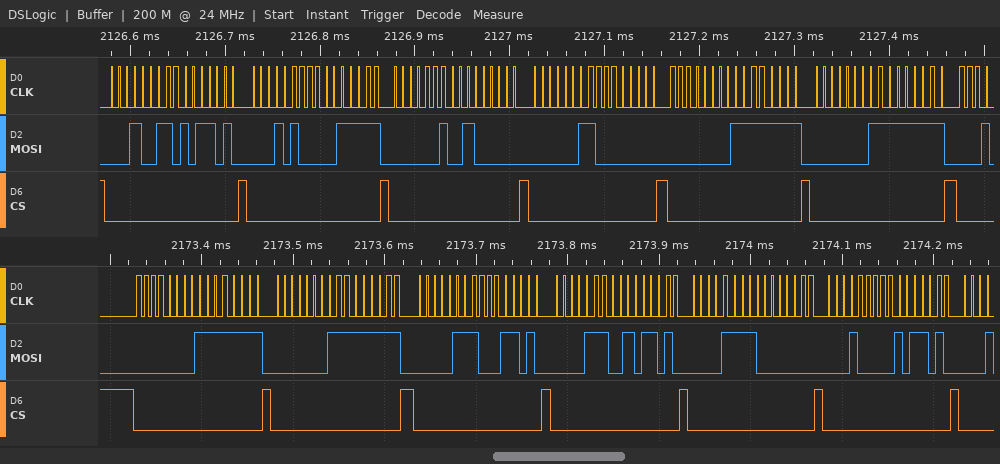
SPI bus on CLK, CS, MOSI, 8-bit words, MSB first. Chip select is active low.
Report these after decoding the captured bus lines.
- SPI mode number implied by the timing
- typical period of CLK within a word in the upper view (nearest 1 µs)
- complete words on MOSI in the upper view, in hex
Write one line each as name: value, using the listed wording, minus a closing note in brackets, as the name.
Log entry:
SPI mode number implied by the timing: 1
typical period of CLK within a word in the upper view: 8 µs
complete words on MOSI in the upper view, in hex: 13, 5A, 14, 1F, 02, 40, 03, 00, 00, FF, 01, FF
